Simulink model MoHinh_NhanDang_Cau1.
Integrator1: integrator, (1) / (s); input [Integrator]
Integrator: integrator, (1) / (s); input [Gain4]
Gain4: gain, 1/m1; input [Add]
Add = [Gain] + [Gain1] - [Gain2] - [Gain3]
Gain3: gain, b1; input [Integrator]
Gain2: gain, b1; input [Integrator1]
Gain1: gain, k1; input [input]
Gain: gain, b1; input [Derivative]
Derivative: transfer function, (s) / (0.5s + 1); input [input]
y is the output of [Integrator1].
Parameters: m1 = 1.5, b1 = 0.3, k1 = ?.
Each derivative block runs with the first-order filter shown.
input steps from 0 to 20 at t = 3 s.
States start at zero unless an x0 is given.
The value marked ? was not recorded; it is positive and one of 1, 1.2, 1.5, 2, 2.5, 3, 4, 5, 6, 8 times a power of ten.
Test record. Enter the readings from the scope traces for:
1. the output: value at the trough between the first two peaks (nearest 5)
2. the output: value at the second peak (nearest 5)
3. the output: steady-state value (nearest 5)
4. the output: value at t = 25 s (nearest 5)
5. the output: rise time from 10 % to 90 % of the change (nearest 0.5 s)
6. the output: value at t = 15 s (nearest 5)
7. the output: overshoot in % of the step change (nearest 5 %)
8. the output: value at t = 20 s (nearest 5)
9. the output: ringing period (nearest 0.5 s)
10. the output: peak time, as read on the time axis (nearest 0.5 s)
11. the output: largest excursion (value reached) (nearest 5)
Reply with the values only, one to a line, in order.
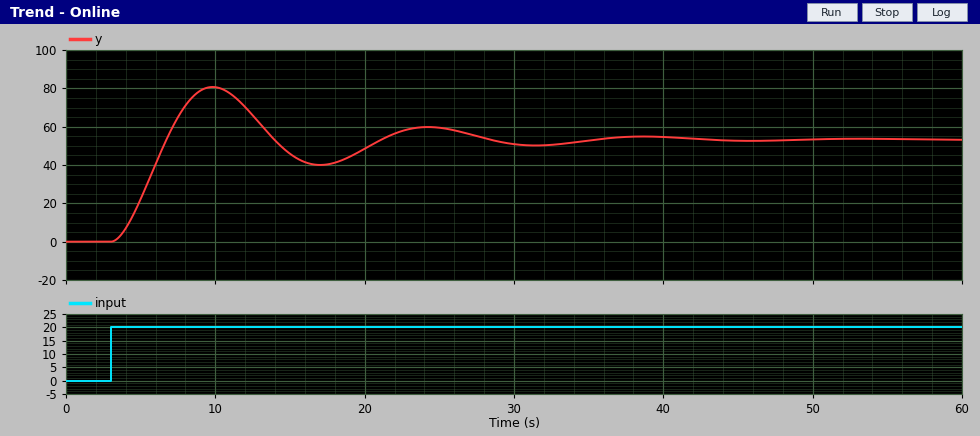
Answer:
40
60
55
60
2.5 s
45
50 %
50
14.5 s
10.0 s
80
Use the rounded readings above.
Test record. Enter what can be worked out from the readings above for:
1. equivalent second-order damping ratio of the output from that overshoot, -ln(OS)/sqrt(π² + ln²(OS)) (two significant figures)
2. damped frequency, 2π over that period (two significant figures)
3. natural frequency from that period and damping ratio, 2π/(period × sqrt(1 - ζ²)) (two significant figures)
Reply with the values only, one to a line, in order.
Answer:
0.22
0.43 rad/s
0.44 rad/s
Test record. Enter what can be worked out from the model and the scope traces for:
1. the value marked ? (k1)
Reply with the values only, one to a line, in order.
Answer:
0.8
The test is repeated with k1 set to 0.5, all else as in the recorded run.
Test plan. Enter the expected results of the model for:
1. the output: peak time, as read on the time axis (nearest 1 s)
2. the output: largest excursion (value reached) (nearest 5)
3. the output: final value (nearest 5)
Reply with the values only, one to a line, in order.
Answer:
10 s
50
35
